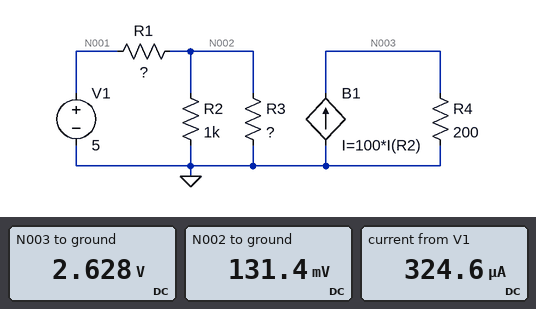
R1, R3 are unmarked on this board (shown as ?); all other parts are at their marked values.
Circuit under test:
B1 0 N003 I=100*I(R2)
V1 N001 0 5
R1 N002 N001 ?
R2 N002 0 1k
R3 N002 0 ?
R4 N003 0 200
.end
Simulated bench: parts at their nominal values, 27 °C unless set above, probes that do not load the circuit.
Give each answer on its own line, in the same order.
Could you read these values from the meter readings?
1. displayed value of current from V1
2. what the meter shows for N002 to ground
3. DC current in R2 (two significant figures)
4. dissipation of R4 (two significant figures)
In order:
324.6 µA
131.4 mV
130 µA
35 mW
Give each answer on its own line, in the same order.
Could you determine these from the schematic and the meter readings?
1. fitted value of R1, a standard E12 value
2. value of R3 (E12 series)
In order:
15 kΩ
680 Ω
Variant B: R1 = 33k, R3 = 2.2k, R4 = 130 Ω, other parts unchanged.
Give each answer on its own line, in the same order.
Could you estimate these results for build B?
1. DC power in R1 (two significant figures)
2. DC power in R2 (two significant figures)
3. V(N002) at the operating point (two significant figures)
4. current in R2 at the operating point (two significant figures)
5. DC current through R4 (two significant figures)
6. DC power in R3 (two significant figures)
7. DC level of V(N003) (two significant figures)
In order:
730 µW
10 µW
100 mV
100 µA
10 mA
4.7 µW
1.3 V
